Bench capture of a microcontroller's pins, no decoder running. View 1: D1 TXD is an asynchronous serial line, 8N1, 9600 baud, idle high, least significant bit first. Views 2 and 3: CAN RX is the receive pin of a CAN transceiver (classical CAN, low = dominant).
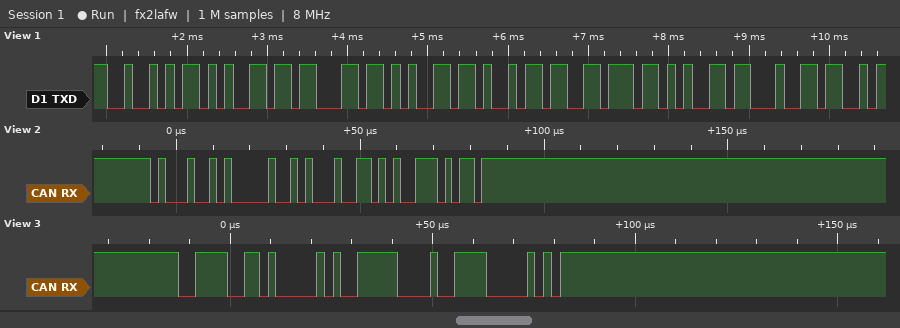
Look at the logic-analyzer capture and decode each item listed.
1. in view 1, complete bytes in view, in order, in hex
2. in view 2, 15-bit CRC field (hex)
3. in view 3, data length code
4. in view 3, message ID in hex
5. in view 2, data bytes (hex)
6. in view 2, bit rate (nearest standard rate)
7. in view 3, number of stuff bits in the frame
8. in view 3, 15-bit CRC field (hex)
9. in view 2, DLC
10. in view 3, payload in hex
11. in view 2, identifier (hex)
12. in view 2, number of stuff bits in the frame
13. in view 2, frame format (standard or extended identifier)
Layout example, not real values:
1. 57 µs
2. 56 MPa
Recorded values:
1. 52 65 63 65 69 76 65 64
2. 0x6A75
3. 1
4. 0x3CD
5. 44
6. 500 kbit/s
7. 3
8. 0x13C0
9. 1
10. 3E
11. 0x44A
12. 1
13. standard
